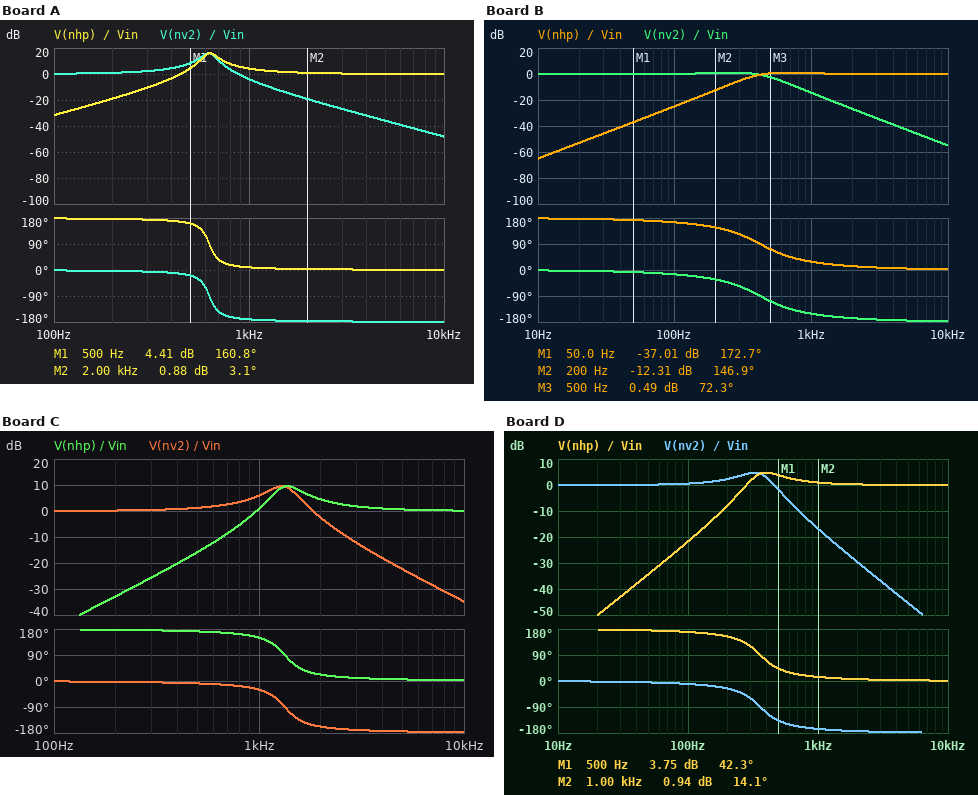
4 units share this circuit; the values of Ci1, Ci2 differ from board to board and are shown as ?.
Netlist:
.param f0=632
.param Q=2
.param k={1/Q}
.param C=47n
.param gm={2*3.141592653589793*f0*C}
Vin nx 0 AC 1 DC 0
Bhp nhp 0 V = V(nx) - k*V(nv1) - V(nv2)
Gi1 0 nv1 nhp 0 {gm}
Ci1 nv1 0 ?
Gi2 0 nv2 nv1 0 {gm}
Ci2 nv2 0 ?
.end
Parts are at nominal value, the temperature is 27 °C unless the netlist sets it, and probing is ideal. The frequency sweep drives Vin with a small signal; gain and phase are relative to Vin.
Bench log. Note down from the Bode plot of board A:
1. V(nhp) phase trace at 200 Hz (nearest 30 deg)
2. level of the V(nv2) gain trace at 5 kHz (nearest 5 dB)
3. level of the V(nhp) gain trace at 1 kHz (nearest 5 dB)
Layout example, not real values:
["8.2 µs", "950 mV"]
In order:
["180 deg", "-35 dB", "5 dB"]
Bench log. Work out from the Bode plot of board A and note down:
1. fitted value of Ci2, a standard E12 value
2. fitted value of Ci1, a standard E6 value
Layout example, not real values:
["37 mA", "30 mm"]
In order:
["15 nF", "150 nF"]
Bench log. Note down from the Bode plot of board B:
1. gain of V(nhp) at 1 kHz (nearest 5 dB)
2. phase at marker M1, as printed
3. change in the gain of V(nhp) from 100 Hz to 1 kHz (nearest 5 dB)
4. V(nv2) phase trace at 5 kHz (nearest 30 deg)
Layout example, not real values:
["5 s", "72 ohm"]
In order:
["0 dB", "172.7 deg", "25 dB", "-180 deg"]
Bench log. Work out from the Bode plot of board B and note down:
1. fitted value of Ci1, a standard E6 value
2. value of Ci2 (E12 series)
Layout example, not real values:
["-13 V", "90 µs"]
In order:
["33 nF", "150 nF"]
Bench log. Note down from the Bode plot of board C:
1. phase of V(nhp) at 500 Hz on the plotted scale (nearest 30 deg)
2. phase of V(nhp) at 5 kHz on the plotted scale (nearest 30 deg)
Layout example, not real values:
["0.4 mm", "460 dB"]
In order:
["180 deg", "0 deg"]
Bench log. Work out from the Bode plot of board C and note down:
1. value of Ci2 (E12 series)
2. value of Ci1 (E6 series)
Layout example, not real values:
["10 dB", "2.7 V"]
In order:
["15 nF", "33 nF"]
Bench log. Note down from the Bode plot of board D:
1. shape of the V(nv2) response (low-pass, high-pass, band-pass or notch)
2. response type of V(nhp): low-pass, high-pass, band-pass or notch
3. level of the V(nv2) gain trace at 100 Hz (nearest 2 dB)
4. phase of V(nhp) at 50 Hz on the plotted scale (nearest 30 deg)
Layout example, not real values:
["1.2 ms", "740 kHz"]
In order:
["low-pass", "high-pass", "0 dB", "180 deg"]
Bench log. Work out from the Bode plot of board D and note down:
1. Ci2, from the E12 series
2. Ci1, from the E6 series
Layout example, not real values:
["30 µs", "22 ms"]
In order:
["100 nF", "68 nF"]
